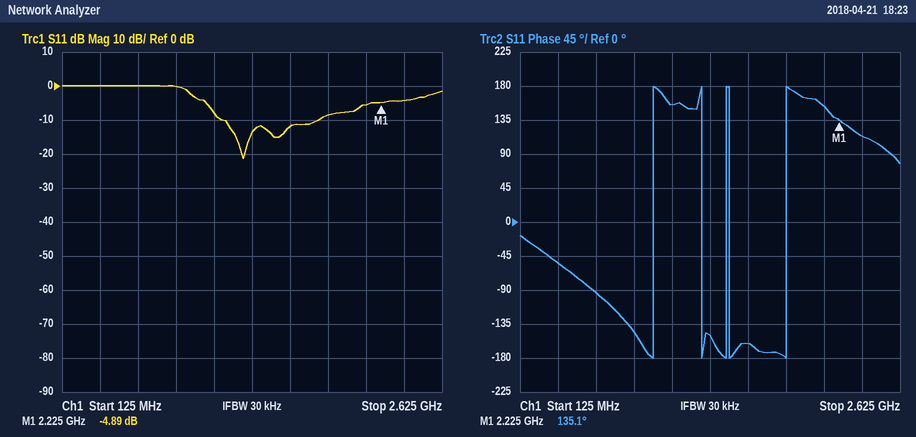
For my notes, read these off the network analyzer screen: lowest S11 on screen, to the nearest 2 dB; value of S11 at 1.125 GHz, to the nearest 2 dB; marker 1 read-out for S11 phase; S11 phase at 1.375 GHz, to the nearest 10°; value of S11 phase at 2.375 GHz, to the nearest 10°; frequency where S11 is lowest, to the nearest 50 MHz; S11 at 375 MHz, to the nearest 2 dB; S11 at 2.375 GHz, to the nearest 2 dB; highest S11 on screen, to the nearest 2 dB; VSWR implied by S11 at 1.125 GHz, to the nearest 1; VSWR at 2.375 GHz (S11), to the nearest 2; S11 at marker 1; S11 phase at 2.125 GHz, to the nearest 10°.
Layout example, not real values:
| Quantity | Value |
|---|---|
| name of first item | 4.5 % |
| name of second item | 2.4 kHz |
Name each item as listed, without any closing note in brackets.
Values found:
| Quantity | Value |
|---|---|
| lowest S11 on screen, to the nearest 2 dB | -22 dB |
| value of S11 at 1.125 GHz, to the nearest 2 dB | -8 dB |
| marker 1 read-out for S11 phase | 135.1° |
| S11 phase at 1.375 GHz, to the nearest 10° | -150° |
| value of S11 phase at 2.375 GHz, to the nearest 10° | 110° |
| frequency where S11 is lowest, to the nearest 50 MHz | 1.30 GHz |
| S11 at 375 MHz, to the nearest 2 dB | 0 dB |
| S11 at 2.375 GHz, to the nearest 2 dB | -4 dB |
| highest S11 on screen, to the nearest 2 dB | 0 dB |
| VSWR implied by S11 at 1.125 GHz, to the nearest 1 | 2 |
| VSWR at 2.375 GHz (S11), to the nearest 2 | 4 |
| S11 at marker 1 | -4.89 dB |
| S11 phase at 2.125 GHz, to the nearest 10° | 150° |
